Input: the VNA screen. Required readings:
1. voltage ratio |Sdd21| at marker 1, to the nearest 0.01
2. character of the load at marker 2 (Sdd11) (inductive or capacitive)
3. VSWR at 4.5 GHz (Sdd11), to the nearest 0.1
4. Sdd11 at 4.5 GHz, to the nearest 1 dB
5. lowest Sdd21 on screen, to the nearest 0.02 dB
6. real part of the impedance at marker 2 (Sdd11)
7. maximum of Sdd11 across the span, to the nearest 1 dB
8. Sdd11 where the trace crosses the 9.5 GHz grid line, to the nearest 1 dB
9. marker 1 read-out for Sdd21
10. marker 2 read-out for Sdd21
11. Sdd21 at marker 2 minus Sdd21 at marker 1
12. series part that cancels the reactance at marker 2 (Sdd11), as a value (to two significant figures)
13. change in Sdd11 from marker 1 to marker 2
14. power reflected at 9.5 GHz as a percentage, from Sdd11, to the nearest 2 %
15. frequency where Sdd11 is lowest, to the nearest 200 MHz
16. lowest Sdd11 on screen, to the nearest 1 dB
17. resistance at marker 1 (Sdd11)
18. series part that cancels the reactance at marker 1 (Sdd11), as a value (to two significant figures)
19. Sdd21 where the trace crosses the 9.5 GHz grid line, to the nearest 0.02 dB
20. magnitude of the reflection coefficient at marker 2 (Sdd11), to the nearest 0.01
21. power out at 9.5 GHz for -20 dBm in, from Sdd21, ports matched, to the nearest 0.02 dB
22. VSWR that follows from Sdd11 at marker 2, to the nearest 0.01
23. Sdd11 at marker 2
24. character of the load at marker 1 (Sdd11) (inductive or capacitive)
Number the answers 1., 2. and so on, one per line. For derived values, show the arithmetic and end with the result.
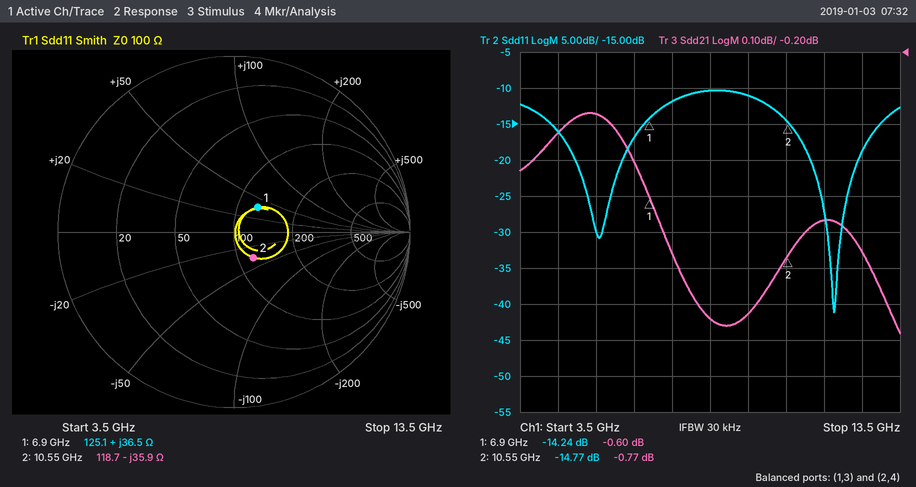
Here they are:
1. 10^(-0.6/20) ≈ 0.93
2. capacitive
3. |Γ| = 10^(-16/20) = 0.1585; VSWR = (1 + 0.1585)/(1 − 0.1585) ≈ 1.4
4. -16 dB
5. -0.98 dB
6. 118.7 Ω
7. -10 dB
8. -11 dB
9. -0.60 dB
10. -0.77 dB
11. -0.77 − (-0.6) = -0.17 dB
12. L = 35.9 Ω/(2π × 10.55 GHz) ≈ 542 pH, so 540 pH to two significant figures
13. -14.77 − (-14.24) = -0.53 dB
14. 10^(-11/10) ≈ 8 %
15. 11.8 GHz
16. -41 dB
17. 125.1 Ω
18. C = 1/(2π × 6.9 GHz × 36.5 Ω) ≈ 632 fF, so 630 fF to two significant figures
19. -0.92 dB
20. 0.18
21. -20 dBm + (-0.92 dB) = -20.92 dBm
22. (1 + 0.1826)/(1 − 0.1826) ≈ 1.45
23. -14.77 dB
24. inductive
